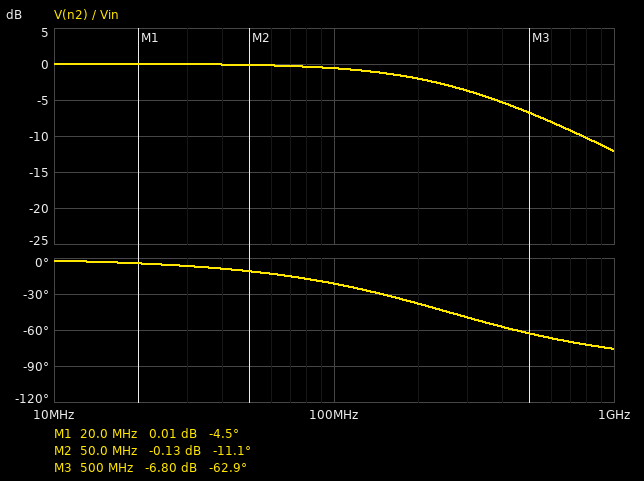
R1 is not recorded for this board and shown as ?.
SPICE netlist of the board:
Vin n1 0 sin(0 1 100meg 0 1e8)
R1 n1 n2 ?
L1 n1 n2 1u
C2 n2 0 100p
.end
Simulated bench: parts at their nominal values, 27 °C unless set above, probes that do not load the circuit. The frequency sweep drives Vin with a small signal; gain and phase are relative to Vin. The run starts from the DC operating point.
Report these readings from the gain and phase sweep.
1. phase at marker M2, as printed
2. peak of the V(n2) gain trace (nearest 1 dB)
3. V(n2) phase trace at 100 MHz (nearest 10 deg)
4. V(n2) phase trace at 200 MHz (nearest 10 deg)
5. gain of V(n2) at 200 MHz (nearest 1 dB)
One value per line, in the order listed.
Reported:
-11.1 deg
0 dB
-20 deg
-40 deg
-2 dB
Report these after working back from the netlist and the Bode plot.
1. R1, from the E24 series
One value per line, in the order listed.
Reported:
6.2 Ω
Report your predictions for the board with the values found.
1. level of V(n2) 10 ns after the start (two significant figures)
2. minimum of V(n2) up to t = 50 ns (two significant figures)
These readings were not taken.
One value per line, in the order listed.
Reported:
-140 mV
-440 mV
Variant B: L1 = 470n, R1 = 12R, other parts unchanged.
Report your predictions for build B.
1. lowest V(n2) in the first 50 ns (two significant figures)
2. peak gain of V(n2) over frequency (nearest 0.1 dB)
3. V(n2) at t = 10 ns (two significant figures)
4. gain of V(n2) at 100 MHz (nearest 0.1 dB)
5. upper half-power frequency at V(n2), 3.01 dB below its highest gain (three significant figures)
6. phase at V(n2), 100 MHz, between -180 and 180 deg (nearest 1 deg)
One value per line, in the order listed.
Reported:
-380 mV
0.2 dB
-220 mV
-1.8 dB
130 MHz
-38 deg
